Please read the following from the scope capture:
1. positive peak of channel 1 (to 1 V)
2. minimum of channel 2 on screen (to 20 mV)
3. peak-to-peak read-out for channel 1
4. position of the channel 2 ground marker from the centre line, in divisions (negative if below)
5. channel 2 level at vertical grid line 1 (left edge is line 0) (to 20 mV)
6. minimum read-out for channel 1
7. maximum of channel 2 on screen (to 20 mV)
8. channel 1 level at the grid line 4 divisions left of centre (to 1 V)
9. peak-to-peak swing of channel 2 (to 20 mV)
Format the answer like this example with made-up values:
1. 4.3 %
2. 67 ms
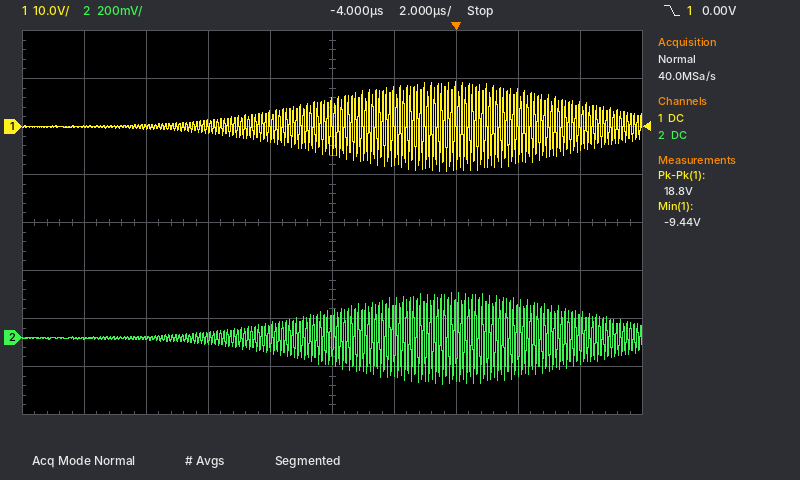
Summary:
1. 9 V
2. -200 mV
3. 18.8 V
4. -2.4 div
5. 0 mV
6. -9.44 V
7. 180 mV
8. 0 V
9. 380 mV
